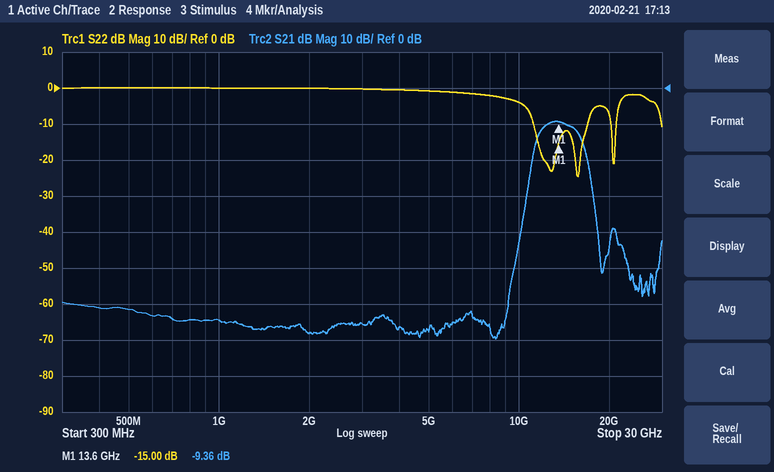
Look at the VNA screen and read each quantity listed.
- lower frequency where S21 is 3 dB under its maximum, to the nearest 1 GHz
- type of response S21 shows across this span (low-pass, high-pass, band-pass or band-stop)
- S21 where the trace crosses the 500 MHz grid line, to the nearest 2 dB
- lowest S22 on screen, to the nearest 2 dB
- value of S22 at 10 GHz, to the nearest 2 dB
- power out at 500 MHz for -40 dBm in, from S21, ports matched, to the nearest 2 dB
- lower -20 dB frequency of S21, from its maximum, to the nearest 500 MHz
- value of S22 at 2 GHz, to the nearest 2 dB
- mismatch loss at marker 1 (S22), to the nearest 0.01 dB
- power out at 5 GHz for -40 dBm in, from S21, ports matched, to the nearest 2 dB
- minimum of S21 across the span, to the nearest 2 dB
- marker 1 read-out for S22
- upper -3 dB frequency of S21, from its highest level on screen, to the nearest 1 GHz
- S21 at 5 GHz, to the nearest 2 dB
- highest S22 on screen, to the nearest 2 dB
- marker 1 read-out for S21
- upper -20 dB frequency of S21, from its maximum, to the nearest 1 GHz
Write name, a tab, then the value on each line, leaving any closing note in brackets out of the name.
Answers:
lower frequency where S21 is 3 dB under its maximum, to the nearest 1 GHz	12 GHz
type of response S21 shows across this span	band-pass
S21 where the trace crosses the 500 MHz grid line, to the nearest 2 dB	-62 dB
lowest S22 on screen, to the nearest 2 dB	-24 dB
value of S22 at 10 GHz, to the nearest 2 dB	-4 dB
power out at 500 MHz for -40 dBm in, from S21, ports matched, to the nearest 2 dB	-102 dBm
lower -20 dB frequency of S21, from its maximum, to the nearest 500 MHz	10.5 GHz
value of S22 at 2 GHz, to the nearest 2 dB	0 dB
mismatch loss at marker 1 (S22), to the nearest 0.01 dB	0.14 dB
power out at 5 GHz for -40 dBm in, from S21, ports matched, to the nearest 2 dB	-108 dBm
minimum of S21 across the span, to the nearest 2 dB	-70 dB
marker 1 read-out for S22	-15.00 dB
upper -3 dB frequency of S21, from its highest level on screen, to the nearest 1 GHz	16 GHz
S21 at 5 GHz, to the nearest 2 dB	-68 dB
highest S22 on screen, to the nearest 2 dB	0 dB
marker 1 read-out for S21	-9.36 dB
upper -20 dB frequency of S21, from its maximum, to the nearest 1 GHz	18 GHz
